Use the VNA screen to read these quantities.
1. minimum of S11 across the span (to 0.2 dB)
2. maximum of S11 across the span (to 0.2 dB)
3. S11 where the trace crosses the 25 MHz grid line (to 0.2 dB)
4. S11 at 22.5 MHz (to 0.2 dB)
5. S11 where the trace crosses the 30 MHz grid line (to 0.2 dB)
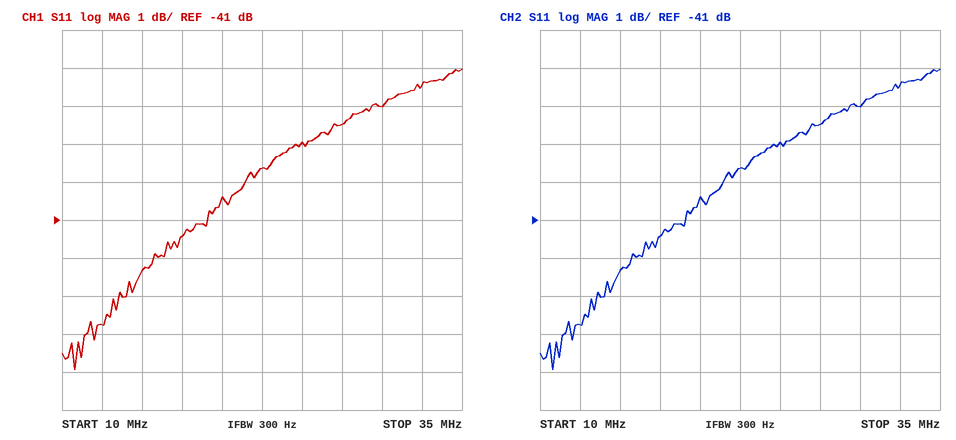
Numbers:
-45.0 dB
-37.0 dB
-39.0 dB
-39.6 dB
-38.0 dB
